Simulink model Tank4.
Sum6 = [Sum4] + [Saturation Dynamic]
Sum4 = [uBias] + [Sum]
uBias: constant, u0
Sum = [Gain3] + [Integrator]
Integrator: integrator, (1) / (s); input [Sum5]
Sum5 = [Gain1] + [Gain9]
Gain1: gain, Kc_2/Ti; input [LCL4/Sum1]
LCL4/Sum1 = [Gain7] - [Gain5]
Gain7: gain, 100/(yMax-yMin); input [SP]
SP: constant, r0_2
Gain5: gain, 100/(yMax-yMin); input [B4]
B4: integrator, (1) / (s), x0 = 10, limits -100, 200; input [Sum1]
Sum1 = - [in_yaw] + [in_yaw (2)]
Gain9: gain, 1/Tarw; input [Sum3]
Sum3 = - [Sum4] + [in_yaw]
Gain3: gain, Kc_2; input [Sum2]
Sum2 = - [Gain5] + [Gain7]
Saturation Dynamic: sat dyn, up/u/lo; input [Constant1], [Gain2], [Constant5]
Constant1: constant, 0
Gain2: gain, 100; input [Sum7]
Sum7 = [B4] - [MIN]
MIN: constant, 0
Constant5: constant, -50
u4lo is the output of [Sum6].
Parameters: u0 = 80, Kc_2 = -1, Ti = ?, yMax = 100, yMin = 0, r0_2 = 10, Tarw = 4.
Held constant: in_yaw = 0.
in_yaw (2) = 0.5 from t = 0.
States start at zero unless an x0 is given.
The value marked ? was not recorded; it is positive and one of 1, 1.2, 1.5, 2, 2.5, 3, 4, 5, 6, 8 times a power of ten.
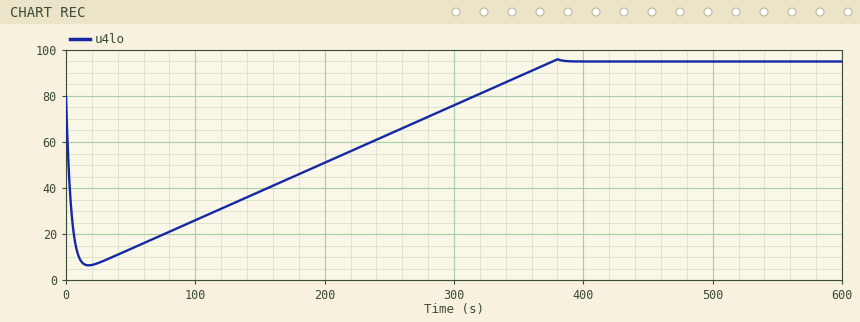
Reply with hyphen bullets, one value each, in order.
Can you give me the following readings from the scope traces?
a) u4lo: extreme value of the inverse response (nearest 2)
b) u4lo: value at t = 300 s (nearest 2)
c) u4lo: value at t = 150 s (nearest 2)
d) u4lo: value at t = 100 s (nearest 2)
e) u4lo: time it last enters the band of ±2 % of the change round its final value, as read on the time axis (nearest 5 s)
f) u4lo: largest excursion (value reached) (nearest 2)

- 6
- 76
- 38
- 26
- 385 s
- 96
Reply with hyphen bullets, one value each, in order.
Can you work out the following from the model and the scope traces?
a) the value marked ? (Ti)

- 8
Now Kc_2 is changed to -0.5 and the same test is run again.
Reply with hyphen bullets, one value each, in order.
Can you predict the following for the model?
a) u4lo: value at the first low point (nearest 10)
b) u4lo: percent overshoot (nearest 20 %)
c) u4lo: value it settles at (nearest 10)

- 0
- 140 %
- 50
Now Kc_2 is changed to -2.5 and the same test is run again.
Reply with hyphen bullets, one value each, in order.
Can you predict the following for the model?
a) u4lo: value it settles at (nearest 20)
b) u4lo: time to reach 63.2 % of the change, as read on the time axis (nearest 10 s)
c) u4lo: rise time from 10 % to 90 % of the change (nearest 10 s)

- 240
- 280 s
- 200 s
